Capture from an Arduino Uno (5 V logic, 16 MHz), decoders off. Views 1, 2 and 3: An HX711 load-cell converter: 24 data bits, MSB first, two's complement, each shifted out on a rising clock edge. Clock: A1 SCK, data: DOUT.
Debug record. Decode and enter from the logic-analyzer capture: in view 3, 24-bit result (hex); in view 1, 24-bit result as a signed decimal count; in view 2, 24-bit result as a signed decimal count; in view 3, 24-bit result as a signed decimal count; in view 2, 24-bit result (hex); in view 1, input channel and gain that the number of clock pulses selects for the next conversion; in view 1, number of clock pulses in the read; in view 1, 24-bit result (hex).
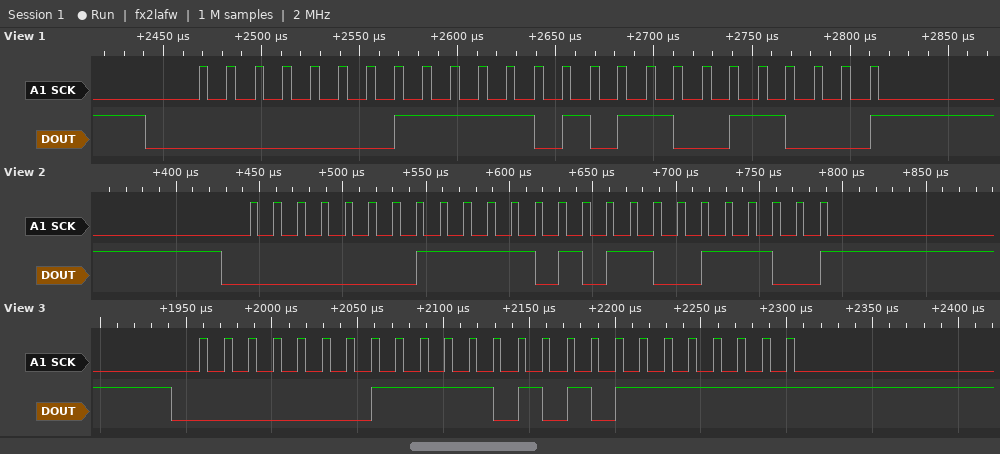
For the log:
0x01F57F
128408
128412
128383
0x01F59C
channel A, gain 128
25
0x01F598
